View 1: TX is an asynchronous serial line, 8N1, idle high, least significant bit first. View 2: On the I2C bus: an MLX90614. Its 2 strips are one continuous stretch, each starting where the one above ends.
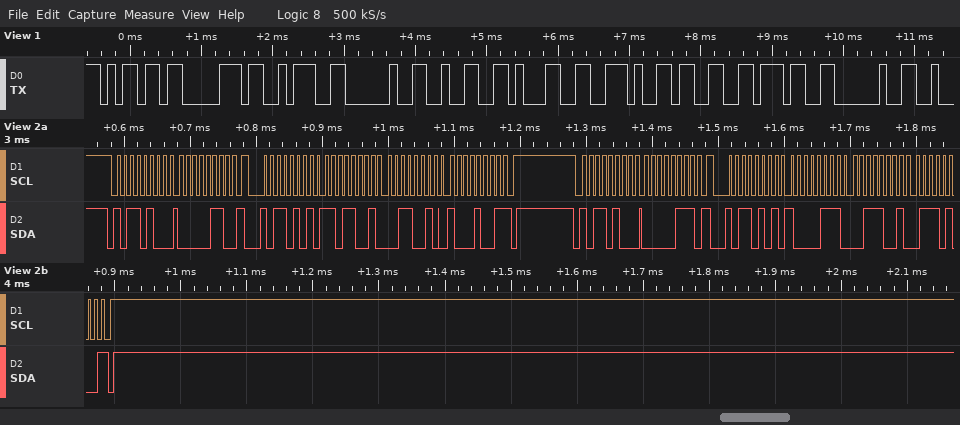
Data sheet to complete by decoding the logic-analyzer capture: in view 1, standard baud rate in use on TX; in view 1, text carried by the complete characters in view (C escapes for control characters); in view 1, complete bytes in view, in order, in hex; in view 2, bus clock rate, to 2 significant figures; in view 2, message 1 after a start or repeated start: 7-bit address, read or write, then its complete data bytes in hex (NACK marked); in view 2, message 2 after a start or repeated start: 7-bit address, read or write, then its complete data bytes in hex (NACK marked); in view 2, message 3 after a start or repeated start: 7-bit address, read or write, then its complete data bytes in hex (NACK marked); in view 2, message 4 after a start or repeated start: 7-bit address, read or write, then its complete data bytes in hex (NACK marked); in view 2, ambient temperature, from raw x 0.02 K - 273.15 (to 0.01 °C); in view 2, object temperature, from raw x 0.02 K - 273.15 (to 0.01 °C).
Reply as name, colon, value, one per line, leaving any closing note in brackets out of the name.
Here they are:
in view 1, standard baud rate in use on TX: 9600 baud
in view 1, text carried by the complete characters in view: "mp: 21.37 "
in view 1, complete bytes in view, in order, in hex: 6D 70 3A 20 32 31 2E 33 37 20
in view 2, bus clock rate, to 2 significant figures: 100 kHz
in view 2, message 1 after a start or repeated start: 7-bit address, read or write, then its complete data bytes in hex: 0x5A write: 06
in view 2, message 2 after a start or repeated start: 7-bit address, read or write, then its complete data bytes in hex: 0x5A read: D9 32 89 NACK
in view 2, message 3 after a start or repeated start: 7-bit address, read or write, then its complete data bytes in hex: 0x5A write: 07
in view 2, message 4 after a start or repeated start: 7-bit address, read or write, then its complete data bytes in hex: 0x5A read: 87 39 74 NACK
in view 2, ambient temperature, from raw x 0.02 K - 273.15: -12.81 °C
in view 2, object temperature, from raw x 0.02 K - 273.15: 21.39 °C
